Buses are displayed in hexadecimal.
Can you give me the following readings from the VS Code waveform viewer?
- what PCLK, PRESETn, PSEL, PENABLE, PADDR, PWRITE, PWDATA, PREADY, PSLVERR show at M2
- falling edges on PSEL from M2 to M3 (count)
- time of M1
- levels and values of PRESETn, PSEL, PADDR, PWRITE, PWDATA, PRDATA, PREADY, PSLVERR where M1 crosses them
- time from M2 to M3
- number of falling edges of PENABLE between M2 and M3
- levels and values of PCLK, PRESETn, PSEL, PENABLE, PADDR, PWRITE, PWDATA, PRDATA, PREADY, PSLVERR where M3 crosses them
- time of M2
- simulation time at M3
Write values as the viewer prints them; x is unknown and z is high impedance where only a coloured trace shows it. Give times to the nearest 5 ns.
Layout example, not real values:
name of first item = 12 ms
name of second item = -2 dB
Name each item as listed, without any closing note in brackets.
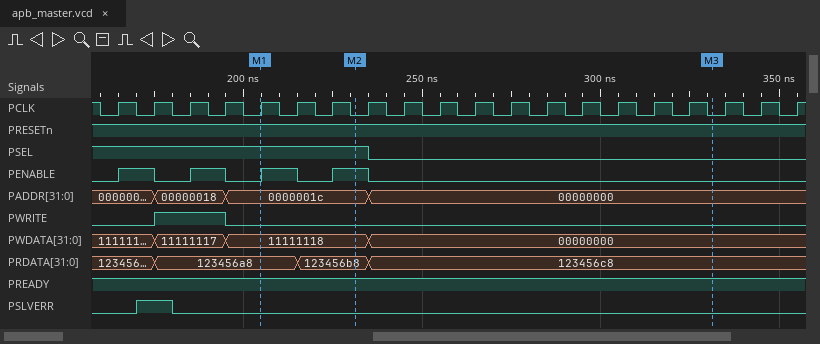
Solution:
what PCLK, PRESETn, PSEL, PENABLE, PADDR, PWRITE, PWDATA, PREADY, PSLVERR show at M2 = PCLK=0, PRESETn=1, PSEL=1, PENABLE=1, PADDR=0000001c, PWRITE=0, PWDATA=11111118, PREADY=1, PSLVERR=0
falling edges on PSEL from M2 to M3 = 1
time of M1 = 205 ns
levels and values of PRESETn, PSEL, PADDR, PWRITE, PWDATA, PRDATA, PREADY, PSLVERR where M1 crosses them = PRESETn=1, PSEL=1, PADDR=0000001c, PWRITE=0, PWDATA=11111118, PRDATA=123456a8, PREADY=1, PSLVERR=0
time from M2 to M3 = 100 ns
number of falling edges of PENABLE between M2 and M3 = 1
levels and values of PCLK, PRESETn, PSEL, PENABLE, PADDR, PWRITE, PWDATA, PRDATA, PREADY, PSLVERR where M3 crosses them = PCLK=0, PRESETn=1, PSEL=0, PENABLE=0, PADDR=00000000, PWRITE=0, PWDATA=00000000, PRDATA=123456c8, PREADY=1, PSLVERR=0
time of M2 = 230 ns
simulation time at M3 = 330 ns
